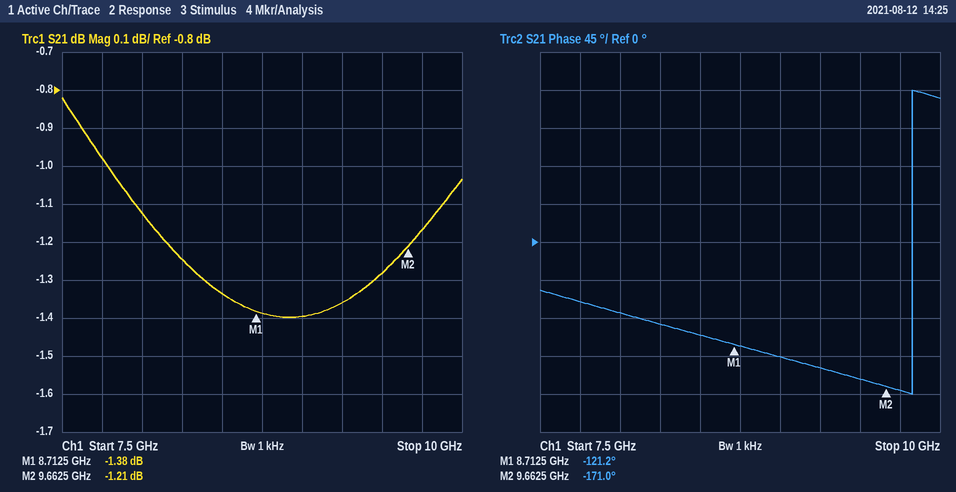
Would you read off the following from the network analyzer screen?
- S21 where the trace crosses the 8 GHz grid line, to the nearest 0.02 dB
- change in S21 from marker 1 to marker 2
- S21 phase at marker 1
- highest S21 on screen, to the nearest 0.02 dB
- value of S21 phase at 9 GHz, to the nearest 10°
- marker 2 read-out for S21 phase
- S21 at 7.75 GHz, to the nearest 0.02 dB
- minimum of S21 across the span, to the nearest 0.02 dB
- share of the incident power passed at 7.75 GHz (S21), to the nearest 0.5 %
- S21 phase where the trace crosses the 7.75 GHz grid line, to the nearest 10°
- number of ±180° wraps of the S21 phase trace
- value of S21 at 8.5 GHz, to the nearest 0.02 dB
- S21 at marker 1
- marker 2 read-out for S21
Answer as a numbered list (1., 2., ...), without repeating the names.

1. -1.12 dB
2. 0.17 dB
3. -121.2°
4. -0.82 dB
5. -140°
6. -171.0°
7. -0.98 dB
8. -1.40 dB
9. 80.0 %
10. -70°
11. 1
12. -1.34 dB
13. -1.38 dB
14. -1.21 dB
